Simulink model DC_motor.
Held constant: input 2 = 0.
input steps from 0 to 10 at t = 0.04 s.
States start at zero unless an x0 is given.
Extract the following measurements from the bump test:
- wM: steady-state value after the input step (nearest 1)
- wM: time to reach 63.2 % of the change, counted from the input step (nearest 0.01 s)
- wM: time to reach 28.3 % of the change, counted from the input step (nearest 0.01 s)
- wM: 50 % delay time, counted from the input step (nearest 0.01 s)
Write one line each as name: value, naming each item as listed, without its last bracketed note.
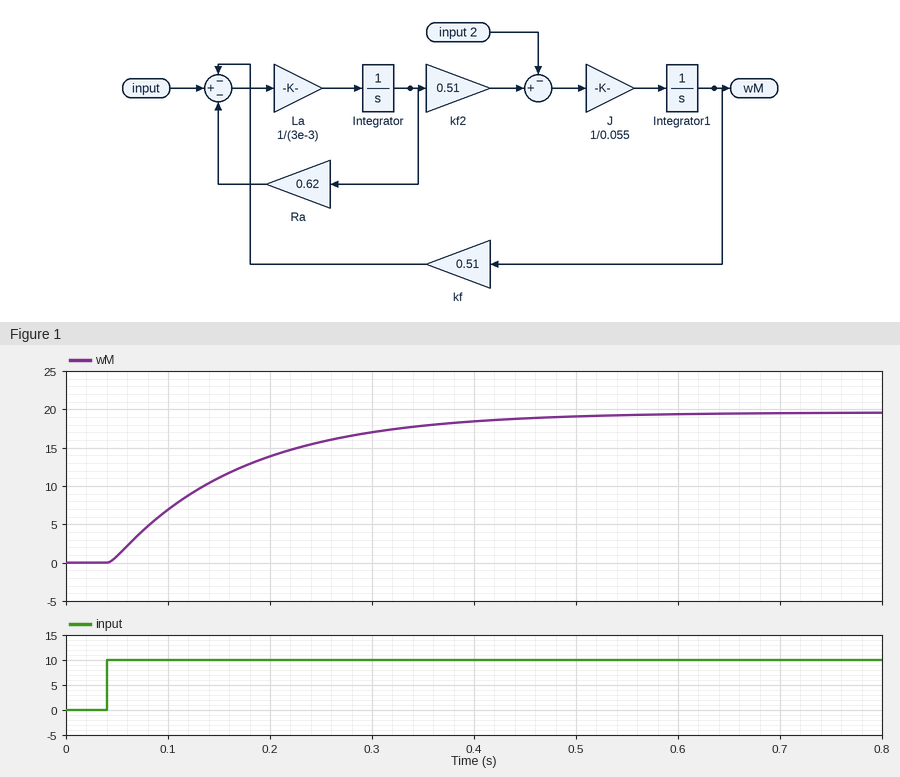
wM: steady-state value after the input step: 20
wM: time to reach 63.2 % of the change, counted from the input step: 0.13 s
wM: time to reach 28.3 % of the change, counted from the input step: 0.05 s
wM: 50 % delay time, counted from the input step: 0.09 s
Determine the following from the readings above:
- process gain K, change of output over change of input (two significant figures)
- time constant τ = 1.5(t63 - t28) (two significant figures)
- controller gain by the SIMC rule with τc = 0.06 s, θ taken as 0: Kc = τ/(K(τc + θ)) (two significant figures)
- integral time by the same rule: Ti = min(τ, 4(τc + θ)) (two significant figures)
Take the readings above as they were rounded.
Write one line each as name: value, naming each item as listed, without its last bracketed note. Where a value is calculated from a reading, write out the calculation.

process gain K, change of output over change of input: (20 - 0) / 10 = 2.0
time constant τ = 1.5(t63 - t28): 1.5 × (0.13 - 0.05) = 0.12 s
controller gain by the SIMC rule with τc = 0.06 s, θ taken as 0: Kc = τ/(K(τc + θ)): 0.12 / (2 × (0.06 + 0)) = 1.0
integral time by the same rule: Ti = min(τ, 4(τc + θ)): min(0.12, 4 × (0.06 + 0)) = 0.12 s
